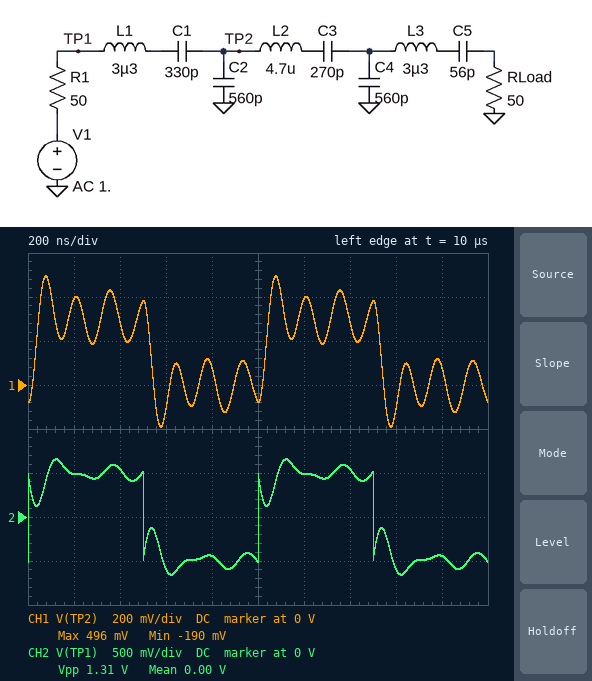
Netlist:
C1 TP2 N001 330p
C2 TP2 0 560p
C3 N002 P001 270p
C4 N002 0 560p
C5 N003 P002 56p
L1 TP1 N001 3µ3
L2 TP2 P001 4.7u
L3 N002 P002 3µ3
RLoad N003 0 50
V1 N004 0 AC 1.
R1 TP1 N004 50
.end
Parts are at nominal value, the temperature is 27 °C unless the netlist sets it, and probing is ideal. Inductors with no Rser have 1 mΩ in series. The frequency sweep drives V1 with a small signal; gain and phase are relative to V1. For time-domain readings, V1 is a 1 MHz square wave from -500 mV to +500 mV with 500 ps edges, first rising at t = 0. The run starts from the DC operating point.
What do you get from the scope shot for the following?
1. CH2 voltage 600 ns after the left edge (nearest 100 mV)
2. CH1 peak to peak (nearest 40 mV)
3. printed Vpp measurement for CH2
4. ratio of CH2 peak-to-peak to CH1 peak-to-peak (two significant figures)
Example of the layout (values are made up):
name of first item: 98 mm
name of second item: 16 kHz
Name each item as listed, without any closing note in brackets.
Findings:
CH2 voltage 600 ns after the left edge: -600 mV
CH1 peak to peak: 680 mV
printed Vpp measurement for CH2: 1.31 V
ratio of CH2 peak-to-peak to CH1 peak-to-peak: 1.9
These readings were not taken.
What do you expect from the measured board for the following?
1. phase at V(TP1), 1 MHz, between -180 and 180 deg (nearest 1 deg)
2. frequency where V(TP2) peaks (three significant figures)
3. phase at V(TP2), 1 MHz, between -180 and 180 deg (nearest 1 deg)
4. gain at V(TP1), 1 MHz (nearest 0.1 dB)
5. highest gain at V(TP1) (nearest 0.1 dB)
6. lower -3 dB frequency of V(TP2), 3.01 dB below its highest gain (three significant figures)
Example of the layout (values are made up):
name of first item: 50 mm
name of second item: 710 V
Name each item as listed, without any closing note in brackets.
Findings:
phase at V(TP1), 1 MHz, between -180 and 180 deg: -4 deg
frequency where V(TP2) peaks: 6.76 MHz
phase at V(TP2), 1 MHz, between -180 and 180 deg: -4 deg
gain at V(TP1), 1 MHz: 0 dB
highest gain at V(TP1): 0 dB
lower -3 dB frequency of V(TP2), 3.01 dB below its highest gain: 6.30 MHz
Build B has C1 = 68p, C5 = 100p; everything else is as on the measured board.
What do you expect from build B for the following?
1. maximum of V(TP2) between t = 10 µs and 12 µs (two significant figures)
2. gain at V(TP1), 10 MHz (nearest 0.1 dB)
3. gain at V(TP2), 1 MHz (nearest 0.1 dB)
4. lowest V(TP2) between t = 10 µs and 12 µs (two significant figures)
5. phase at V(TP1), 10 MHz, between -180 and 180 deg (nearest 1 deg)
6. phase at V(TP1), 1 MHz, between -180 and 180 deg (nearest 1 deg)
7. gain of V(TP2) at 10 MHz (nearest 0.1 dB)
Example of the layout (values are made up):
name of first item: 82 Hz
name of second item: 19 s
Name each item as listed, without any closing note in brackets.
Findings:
maximum of V(TP2) between t = 10 µs and 12 µs: 170 mV
gain at V(TP1), 10 MHz: -2.3 dB
gain at V(TP2), 1 MHz: -21.6 dB
lowest V(TP2) between t = 10 µs and 12 µs: -85 mV
phase at V(TP1), 10 MHz, between -180 and 180 deg: -40 deg
phase at V(TP1), 1 MHz, between -180 and 180 deg: -1 deg
gain of V(TP2) at 10 MHz: -7.5 dB
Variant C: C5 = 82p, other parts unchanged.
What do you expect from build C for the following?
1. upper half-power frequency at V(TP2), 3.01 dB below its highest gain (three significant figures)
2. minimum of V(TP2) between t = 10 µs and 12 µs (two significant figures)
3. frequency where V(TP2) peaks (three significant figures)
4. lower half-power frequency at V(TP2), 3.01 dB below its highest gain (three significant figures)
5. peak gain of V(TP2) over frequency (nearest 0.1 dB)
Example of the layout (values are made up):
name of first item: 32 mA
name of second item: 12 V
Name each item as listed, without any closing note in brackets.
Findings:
upper half-power frequency at V(TP2), 3.01 dB below its highest gain: 7.29 MHz
minimum of V(TP2) between t = 10 µs and 12 µs: -180 mV
frequency where V(TP2) peaks: 6.73 MHz
lower half-power frequency at V(TP2), 3.01 dB below its highest gain: 6.24 MHz
peak gain of V(TP2) over frequency: 4.0 dB
